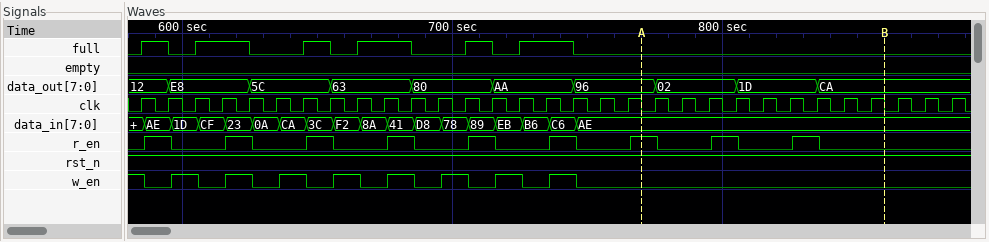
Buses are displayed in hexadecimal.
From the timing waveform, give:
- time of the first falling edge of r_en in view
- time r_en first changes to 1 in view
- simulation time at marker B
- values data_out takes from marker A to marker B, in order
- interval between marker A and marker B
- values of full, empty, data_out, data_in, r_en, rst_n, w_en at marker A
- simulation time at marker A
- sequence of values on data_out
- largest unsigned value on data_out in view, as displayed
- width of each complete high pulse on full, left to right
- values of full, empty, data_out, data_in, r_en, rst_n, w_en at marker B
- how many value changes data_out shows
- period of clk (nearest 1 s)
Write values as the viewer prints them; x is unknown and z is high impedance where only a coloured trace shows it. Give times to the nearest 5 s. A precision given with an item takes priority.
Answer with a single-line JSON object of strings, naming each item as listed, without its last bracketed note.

{"time of the first falling edge of r_en in view": "595 s", "time r_en first changes to 1 in view": "585 s", "simulation time at marker B": "860 s", "values data_out takes from marker A to marker B, in order": "96, 02, 1D, CA", "interval between marker A and marker B": "90 s", "values of full, empty, data_out, data_in, r_en, rst_n, w_en at marker A": "full=0, empty=0, data_out=96, data_in=AE, r_en=1, rst_n=1, w_en=0", "simulation time at marker A": "770 s", "sequence of values on data_out": "12, E8, 5C, 63, 80, AA, 96, 02, 1D, CA", "largest unsigned value on data_out in view, as displayed": "E8", "width of each complete high pulse on full, left to right": "10 s, 20 s, 10 s, 20 s, 10 s, 20 s", "values of full, empty, data_out, data_in, r_en, rst_n, w_en at marker B": "full=0, empty=0, data_out=CA, data_in=AE, r_en=0, rst_n=1, w_en=0", "how many value changes data_out shows": "9", "period of clk": "10 s"}
